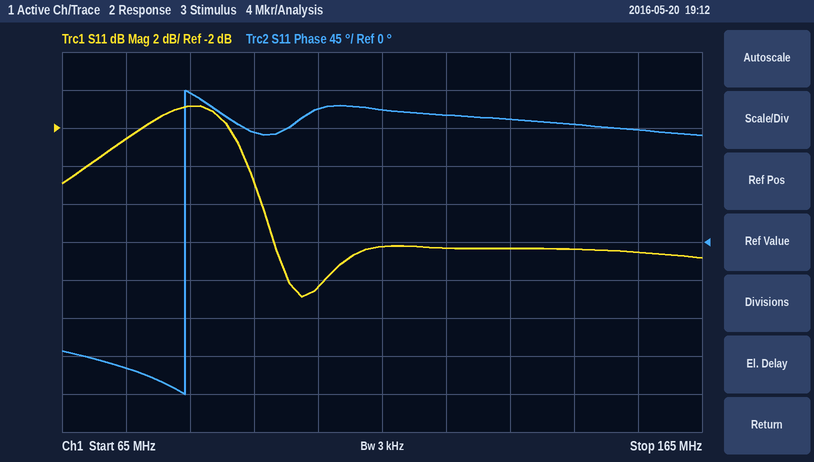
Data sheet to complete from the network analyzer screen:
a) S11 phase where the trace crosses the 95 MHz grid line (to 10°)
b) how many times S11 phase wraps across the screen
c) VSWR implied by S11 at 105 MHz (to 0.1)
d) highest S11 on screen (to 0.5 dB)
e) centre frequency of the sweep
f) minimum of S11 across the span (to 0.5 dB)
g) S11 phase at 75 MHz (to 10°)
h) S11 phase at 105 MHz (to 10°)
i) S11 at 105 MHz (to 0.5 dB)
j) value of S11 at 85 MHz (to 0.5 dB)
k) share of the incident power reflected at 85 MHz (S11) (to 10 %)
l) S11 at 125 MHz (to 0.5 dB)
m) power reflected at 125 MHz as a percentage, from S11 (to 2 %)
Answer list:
130°
1
1.9
-1.0 dB
115 MHz
-11.0 dB
-150°
160°
-10.5 dB
-1.0 dB
80 %
-8.5 dB
14 %
